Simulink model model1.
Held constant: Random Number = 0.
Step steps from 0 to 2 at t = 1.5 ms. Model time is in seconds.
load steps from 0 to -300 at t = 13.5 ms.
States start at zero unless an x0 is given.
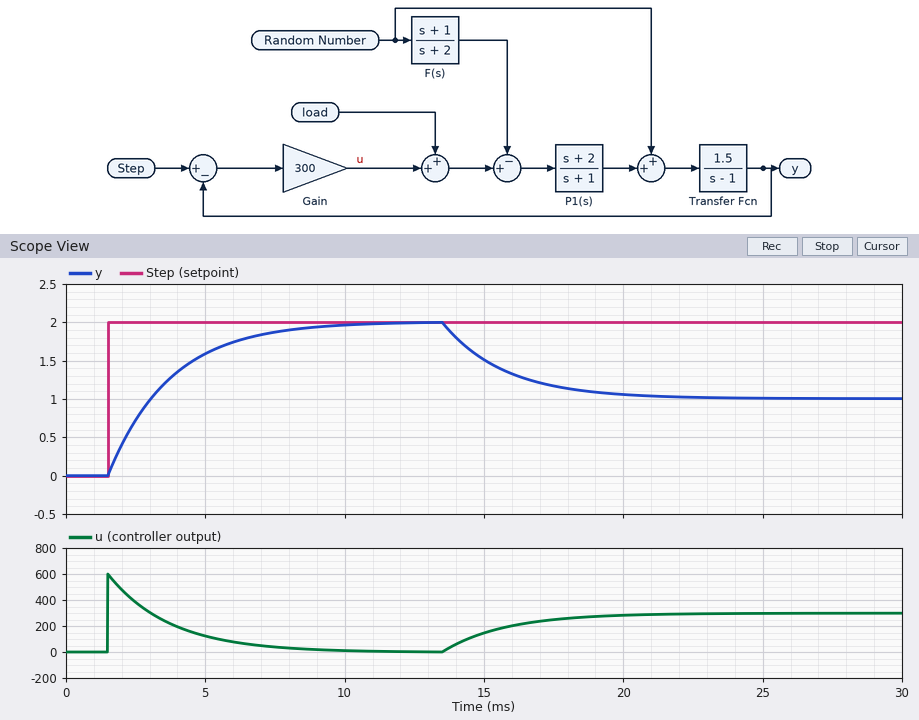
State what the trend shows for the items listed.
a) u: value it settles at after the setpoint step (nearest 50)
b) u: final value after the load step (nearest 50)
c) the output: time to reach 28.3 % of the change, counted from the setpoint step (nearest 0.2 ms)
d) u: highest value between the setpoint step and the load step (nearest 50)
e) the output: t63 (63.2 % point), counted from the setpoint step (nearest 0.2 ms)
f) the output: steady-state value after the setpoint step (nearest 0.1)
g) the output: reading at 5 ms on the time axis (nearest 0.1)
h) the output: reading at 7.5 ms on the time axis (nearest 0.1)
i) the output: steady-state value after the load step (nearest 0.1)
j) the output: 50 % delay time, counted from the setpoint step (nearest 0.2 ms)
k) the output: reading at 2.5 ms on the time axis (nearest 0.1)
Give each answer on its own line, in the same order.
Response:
0
300
0.8 ms
600
2.2 ms
2.0
1.6
1.9
1.0
1.6 ms
0.7
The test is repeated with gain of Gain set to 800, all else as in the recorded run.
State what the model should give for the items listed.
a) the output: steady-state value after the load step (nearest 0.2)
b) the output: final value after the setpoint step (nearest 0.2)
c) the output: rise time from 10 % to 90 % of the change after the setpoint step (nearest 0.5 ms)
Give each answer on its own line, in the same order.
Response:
1.6
2.0
2.0 ms
